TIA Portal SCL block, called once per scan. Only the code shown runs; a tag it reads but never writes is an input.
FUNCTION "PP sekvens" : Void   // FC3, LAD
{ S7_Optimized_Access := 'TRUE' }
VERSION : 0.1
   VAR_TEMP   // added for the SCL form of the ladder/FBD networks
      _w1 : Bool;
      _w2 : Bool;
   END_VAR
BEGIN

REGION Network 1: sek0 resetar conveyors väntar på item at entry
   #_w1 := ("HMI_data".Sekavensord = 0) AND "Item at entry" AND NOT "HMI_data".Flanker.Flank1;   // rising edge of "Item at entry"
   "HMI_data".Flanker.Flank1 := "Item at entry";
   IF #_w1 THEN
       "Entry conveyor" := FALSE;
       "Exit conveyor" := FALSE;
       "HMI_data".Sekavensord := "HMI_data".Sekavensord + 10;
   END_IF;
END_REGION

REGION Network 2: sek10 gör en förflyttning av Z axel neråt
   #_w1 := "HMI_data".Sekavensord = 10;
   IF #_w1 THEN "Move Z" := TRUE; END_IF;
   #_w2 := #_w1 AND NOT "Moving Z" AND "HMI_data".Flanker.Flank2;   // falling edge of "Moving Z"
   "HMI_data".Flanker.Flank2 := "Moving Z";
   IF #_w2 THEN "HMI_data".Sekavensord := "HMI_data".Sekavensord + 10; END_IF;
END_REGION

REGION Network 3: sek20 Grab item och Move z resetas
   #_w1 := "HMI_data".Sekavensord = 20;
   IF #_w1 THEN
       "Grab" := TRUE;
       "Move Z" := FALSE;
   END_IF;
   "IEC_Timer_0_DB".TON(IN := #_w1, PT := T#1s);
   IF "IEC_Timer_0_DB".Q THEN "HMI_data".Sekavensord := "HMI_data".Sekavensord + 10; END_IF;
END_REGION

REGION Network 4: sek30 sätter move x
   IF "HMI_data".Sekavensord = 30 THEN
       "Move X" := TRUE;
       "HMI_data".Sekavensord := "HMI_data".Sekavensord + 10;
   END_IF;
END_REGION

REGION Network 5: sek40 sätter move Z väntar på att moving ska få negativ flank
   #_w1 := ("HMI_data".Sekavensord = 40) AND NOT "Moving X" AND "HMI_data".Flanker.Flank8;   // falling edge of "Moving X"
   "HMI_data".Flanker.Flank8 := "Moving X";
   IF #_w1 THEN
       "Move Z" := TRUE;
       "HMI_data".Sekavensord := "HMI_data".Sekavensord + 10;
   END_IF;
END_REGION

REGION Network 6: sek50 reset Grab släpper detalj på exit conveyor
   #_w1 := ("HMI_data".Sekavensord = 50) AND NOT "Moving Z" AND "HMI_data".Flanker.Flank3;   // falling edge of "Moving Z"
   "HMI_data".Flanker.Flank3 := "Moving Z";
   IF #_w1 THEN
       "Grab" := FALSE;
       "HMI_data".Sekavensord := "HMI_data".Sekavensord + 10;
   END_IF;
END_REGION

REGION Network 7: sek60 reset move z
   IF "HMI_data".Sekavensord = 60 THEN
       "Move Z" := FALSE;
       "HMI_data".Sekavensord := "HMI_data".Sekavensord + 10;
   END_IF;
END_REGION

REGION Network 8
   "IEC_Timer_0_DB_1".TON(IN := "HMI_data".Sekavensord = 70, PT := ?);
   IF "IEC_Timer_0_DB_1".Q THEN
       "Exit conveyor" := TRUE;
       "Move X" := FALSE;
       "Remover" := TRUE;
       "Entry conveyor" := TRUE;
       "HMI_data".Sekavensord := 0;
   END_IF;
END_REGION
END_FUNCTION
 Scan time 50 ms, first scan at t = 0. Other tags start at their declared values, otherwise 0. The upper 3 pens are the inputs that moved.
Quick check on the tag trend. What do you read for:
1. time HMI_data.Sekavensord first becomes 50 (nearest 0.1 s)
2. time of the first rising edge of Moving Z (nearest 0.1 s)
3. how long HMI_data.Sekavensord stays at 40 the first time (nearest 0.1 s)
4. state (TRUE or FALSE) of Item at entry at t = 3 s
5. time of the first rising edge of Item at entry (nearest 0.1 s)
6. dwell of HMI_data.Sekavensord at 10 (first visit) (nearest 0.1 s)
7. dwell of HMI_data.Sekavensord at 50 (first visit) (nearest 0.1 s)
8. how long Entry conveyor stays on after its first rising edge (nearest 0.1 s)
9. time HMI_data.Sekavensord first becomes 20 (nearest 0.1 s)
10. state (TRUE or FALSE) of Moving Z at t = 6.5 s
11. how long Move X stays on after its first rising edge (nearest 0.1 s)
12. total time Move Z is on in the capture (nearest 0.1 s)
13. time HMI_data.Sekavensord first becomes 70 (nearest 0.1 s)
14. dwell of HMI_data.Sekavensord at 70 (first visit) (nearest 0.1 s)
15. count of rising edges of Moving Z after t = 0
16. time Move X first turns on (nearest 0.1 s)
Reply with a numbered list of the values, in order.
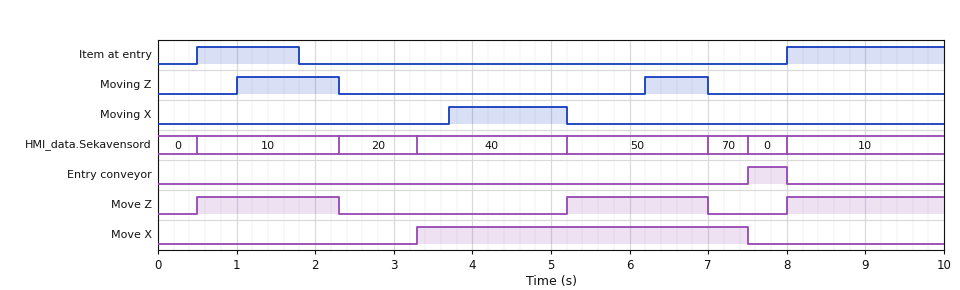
1. 5.2 s
2. 1.0 s
3. 1.9 s
4. FALSE
5. 0.5 s
6. 1.8 s
7. 1.8 s
8. 0.5 s
9. 2.3 s
10. TRUE
11. 4.2 s
12. 5.6 s
13. 7.0 s
14. 0.5 s
15. 2
16. 3.3 s
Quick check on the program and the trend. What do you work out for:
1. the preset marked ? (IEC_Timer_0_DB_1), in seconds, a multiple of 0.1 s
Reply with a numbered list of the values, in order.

1. 0.5 s
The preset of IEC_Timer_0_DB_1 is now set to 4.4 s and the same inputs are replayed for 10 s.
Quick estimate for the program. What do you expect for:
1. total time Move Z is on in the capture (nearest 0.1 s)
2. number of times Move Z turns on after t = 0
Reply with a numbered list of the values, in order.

1. 3.6 s
2. 2
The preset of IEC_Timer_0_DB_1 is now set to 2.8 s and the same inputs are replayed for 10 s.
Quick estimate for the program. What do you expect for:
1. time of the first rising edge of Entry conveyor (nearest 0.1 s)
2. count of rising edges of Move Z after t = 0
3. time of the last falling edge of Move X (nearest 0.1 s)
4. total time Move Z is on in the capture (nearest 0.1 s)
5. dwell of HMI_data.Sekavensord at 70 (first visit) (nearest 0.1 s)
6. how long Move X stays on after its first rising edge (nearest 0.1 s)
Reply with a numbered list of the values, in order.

1. 9.8 s
2. 2
3. 9.8 s
4. 3.6 s
5. 2.8 s
6. 6.5 s
